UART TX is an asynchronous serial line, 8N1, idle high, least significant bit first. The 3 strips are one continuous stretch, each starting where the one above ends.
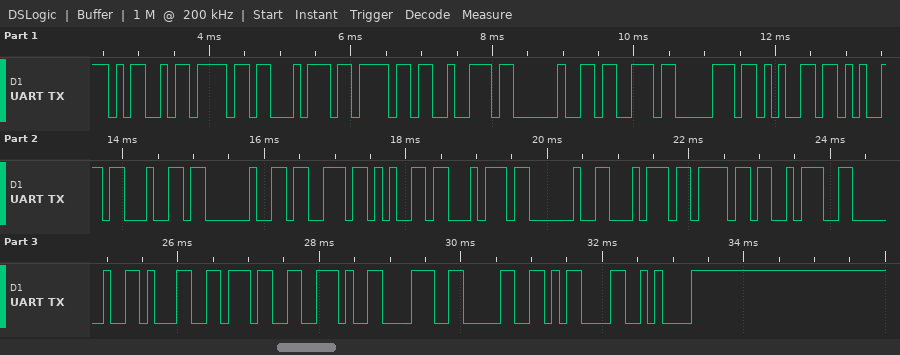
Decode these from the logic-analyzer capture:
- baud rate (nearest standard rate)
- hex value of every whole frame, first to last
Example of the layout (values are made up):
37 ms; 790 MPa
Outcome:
9600 baud; 4D 6F 74 6F 72 20 73 70 65 65 64 20 73 65 74 20 74 6F 3A 20 31 37 2E 38 30 0D 0A
